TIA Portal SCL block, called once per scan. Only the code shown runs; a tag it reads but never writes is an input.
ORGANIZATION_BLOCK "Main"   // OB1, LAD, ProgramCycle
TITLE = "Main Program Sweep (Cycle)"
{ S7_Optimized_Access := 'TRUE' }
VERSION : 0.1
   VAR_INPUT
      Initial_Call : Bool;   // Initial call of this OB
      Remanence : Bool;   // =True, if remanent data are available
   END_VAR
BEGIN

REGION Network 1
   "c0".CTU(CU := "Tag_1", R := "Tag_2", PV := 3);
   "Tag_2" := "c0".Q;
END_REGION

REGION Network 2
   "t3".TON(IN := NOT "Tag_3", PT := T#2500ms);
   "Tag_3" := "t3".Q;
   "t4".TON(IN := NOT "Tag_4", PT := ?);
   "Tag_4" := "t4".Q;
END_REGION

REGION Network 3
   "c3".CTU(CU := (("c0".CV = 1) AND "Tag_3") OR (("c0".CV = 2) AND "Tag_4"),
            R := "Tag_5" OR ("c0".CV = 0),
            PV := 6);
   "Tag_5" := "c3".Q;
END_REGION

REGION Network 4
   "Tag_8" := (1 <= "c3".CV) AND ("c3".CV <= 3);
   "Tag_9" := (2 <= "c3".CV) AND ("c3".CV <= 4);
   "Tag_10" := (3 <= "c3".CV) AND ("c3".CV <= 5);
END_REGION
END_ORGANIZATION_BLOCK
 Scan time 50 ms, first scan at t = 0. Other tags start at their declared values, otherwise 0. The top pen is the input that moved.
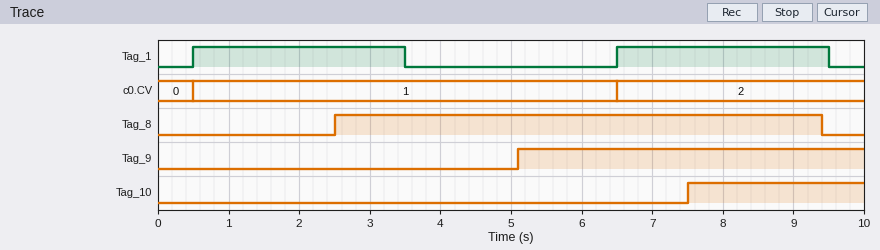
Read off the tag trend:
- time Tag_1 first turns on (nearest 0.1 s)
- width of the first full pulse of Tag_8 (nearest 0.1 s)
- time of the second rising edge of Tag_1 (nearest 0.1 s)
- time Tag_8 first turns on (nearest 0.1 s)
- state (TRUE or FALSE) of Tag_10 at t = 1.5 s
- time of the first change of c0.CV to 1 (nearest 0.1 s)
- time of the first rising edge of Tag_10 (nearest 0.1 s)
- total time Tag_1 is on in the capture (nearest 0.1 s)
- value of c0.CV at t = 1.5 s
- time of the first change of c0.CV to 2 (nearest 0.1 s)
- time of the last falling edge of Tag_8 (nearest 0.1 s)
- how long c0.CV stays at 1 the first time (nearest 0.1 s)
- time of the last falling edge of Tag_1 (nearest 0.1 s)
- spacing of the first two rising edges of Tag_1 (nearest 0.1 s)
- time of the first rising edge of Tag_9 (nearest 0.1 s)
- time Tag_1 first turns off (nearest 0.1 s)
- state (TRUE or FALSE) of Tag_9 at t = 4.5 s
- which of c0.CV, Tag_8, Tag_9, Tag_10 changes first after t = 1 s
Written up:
0.5 s
6.9 s
6.5 s
2.5 s
FALSE
0.5 s
7.5 s
6.0 s
1
6.5 s
9.4 s
6.0 s
9.5 s
6.0 s
5.1 s
3.5 s
FALSE
Tag_8
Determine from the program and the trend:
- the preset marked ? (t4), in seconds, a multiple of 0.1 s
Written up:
1.8 s
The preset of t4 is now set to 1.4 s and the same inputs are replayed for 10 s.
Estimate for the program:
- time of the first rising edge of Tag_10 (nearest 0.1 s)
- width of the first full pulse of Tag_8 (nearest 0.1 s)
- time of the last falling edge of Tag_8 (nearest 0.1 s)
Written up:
7.4 s
6.4 s
8.9 s
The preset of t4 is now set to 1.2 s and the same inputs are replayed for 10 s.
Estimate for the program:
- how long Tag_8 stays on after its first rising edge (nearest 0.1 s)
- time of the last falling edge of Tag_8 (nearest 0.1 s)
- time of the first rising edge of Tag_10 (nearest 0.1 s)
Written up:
6.5 s
9.0 s
7.7 s
